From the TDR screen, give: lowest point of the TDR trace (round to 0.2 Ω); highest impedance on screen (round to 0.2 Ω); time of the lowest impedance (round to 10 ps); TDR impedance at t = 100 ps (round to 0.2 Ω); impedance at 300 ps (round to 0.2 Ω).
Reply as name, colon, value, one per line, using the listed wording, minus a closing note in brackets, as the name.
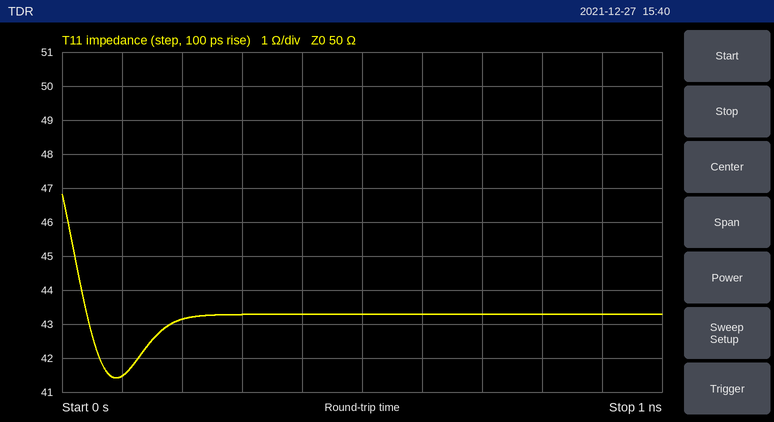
lowest point of the TDR trace: 41.4 Ω
highest impedance on screen: 46.8 Ω
time of the lowest impedance: 90 ps
TDR impedance at t = 100 ps: 41.4 Ω
impedance at 300 ps: 43.2 Ω
